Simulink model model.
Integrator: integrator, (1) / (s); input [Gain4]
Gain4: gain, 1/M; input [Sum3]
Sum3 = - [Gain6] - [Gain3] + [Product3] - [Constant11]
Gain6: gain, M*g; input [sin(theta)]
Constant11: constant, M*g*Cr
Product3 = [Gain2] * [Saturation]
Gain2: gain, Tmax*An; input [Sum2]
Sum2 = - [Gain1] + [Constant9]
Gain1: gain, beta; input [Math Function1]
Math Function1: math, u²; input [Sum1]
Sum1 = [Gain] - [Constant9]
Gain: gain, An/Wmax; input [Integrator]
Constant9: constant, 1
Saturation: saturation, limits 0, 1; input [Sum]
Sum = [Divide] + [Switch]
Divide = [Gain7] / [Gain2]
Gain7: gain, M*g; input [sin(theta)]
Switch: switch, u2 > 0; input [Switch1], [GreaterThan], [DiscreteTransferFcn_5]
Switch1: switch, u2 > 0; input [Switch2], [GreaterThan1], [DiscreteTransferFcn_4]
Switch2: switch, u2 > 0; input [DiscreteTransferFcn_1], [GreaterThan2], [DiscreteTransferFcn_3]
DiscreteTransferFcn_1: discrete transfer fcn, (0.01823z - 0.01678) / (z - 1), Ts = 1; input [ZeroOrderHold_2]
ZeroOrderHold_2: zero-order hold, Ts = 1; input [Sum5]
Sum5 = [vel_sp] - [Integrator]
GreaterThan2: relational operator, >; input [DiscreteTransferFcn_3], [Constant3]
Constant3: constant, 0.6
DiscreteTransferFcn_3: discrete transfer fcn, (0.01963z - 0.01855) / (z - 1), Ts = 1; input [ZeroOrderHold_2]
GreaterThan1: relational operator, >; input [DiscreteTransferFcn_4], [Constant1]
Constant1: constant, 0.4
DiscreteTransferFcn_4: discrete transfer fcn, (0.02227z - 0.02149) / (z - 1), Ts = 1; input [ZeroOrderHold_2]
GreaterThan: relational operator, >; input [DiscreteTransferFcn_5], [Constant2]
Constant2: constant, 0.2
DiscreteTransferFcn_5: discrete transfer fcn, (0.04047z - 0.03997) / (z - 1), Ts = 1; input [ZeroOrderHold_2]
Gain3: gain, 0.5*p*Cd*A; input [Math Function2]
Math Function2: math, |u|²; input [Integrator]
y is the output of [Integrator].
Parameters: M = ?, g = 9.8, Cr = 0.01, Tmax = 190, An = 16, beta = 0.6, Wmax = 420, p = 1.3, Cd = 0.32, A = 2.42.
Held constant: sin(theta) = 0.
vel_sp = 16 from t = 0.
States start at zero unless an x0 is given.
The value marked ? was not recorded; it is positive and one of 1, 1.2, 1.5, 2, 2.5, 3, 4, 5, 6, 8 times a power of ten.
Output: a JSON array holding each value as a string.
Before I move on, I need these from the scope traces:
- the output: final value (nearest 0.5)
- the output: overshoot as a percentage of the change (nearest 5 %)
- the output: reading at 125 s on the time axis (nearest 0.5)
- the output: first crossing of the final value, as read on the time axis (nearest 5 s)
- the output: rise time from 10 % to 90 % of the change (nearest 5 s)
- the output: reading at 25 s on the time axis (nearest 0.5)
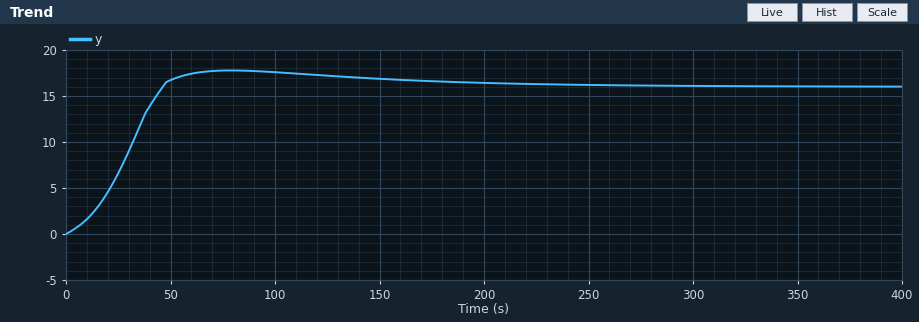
["16.0", "10 %", "17.0", "45 s", "30 s", "6.5"]
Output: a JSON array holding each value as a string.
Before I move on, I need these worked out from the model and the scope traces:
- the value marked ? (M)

["2000"]
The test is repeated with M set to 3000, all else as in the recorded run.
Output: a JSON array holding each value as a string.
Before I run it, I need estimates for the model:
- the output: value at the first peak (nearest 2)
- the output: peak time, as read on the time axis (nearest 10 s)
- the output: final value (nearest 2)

["18", "80 s", "16"]
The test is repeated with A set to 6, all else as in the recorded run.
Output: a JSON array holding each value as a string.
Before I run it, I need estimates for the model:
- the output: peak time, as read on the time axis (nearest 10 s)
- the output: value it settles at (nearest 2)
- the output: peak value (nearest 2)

["50 s", "16", "16"]
